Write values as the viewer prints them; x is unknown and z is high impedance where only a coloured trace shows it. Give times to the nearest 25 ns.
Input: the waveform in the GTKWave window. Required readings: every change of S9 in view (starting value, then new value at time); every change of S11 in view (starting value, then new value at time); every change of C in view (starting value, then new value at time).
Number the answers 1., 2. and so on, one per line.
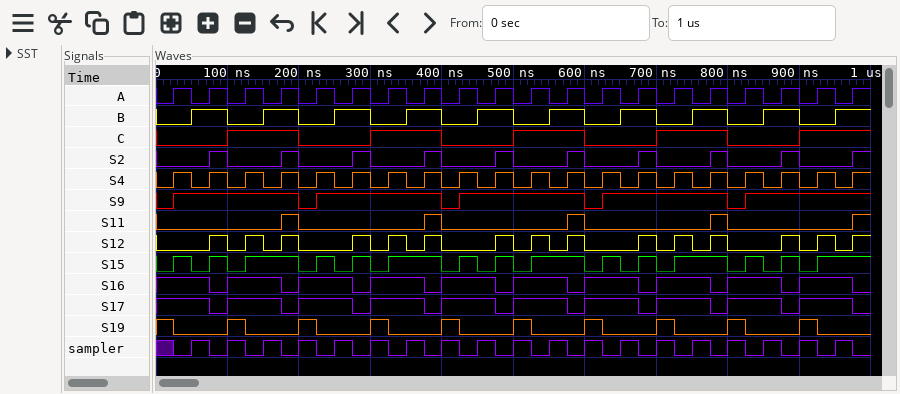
1. 0, 1 at 25 ns, 0 at 200 ns, 1 at 225 ns, 0 at 400 ns, 1 at 425 ns, 0 at 600 ns, 1 at 625 ns, 0 at 800 ns, 1 at 825 ns
2. 0, 1 at 175 ns, 0 at 200 ns, 1 at 375 ns, 0 at 400 ns, 1 at 575 ns, 0 at 600 ns, 1 at 775 ns, 0 at 800 ns, 1 at 975 ns
3. 0, 1 at 100 ns, 0 at 200 ns, 1 at 300 ns, 0 at 400 ns, 1 at 500 ns, 0 at 600 ns, 1 at 700 ns, 0 at 800 ns, 1 at 900 ns
